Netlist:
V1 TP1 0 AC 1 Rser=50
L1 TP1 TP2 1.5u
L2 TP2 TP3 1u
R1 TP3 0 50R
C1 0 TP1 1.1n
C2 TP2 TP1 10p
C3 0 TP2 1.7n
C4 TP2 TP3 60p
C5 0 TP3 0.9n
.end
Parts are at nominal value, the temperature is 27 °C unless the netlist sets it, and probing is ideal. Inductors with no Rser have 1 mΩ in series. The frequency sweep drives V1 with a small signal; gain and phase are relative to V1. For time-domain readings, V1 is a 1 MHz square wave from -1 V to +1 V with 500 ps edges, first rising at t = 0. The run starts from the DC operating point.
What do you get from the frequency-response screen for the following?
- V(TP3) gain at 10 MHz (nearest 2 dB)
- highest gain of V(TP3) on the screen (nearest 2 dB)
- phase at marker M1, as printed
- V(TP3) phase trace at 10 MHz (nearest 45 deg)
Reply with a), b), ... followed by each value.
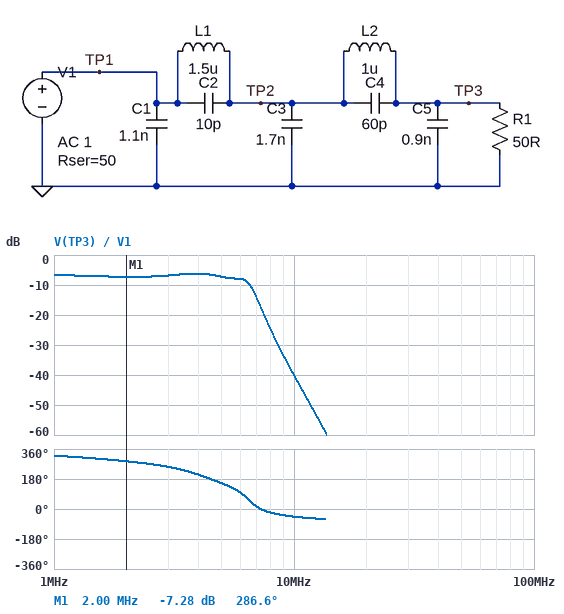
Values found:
a) -40 dB
b) -6 dB
c) 286.6 deg
d) -45 deg
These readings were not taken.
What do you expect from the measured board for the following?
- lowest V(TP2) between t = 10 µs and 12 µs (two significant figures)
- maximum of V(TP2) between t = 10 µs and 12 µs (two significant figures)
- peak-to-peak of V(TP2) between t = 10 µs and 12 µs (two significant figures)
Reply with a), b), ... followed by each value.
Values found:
a) -520 mV
b) 520 mV
c) 1.0 V
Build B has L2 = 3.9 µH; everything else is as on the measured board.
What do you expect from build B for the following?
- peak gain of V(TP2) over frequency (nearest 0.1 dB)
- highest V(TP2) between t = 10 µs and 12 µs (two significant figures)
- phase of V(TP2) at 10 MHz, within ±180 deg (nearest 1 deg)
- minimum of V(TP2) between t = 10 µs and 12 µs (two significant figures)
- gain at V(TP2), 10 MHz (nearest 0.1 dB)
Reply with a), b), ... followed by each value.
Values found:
a) -1.3 dB
b) 770 mV
c) 109 deg
d) -770 mV
e) -29.5 dB
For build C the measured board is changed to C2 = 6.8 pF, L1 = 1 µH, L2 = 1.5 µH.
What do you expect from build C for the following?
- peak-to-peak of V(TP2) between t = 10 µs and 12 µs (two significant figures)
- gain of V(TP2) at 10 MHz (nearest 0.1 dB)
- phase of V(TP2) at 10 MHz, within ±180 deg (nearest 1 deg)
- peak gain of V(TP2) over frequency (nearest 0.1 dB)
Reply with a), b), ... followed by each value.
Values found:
a) 1.1 V
b) -23.4 dB
c) 112 deg
d) -1.9 dB
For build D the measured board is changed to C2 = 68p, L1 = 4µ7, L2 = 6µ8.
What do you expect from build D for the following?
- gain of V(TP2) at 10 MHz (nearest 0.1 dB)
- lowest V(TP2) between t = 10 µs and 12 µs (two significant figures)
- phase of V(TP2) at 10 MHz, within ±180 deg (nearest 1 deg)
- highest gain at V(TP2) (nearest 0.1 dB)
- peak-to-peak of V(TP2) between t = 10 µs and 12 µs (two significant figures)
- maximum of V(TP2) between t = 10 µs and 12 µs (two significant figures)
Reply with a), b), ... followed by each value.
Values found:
a) -53.0 dB
b) -920 mV
c) -74 deg
d) 0.8 dB
e) 1.8 V
f) 920 mV
